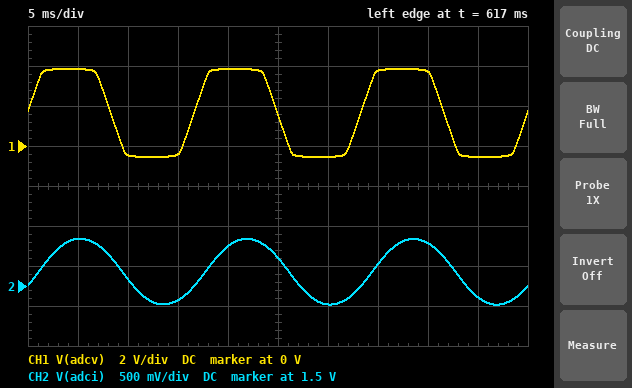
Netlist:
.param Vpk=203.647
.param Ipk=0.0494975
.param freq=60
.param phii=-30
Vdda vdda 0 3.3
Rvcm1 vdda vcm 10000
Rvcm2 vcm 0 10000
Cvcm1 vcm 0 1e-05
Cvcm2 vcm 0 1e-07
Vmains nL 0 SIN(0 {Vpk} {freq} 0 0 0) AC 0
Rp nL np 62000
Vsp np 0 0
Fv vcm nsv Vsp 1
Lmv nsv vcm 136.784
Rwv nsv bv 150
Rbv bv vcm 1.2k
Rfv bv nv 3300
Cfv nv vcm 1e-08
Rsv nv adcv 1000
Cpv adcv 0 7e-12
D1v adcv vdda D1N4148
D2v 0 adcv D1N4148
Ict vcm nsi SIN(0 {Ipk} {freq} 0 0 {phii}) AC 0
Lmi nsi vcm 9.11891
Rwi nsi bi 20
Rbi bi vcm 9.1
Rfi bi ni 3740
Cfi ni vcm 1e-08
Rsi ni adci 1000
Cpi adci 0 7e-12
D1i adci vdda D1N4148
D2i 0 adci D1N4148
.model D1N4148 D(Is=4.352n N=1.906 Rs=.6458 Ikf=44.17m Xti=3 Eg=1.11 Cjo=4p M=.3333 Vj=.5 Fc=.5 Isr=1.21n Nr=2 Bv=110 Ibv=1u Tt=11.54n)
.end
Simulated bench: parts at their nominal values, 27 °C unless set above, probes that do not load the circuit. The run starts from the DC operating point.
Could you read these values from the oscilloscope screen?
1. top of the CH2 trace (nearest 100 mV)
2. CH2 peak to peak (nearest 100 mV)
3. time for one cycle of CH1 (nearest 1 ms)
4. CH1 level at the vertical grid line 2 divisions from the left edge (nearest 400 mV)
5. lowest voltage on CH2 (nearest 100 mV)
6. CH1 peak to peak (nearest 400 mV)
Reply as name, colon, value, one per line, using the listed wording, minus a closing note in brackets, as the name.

top of the CH2 trace: 2.1 V
CH2 peak to peak: 800 mV
time for one cycle of CH1: 17 ms
CH1 level at the vertical grid line 2 divisions from the left edge: -400 mV
lowest voltage on CH2: 1.3 V
CH1 peak to peak: 4.4 V
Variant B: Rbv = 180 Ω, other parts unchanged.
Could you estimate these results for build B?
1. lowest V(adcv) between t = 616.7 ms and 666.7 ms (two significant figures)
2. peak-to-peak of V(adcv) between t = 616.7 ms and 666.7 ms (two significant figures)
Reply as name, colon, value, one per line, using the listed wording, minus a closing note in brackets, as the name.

lowest V(adcv) between t = 616.7 ms and 666.7 ms: 1.1 V
peak-to-peak of V(adcv) between t = 616.7 ms and 666.7 ms: 1.2 V
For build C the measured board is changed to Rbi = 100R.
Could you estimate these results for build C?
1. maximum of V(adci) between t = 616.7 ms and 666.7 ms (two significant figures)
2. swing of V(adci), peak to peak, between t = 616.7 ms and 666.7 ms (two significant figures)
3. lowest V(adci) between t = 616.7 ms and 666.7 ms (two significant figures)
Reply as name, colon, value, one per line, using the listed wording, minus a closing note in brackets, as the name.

maximum of V(adci) between t = 616.7 ms and 666.7 ms: 3.9 V
swing of V(adci), peak to peak, between t = 616.7 ms and 666.7 ms: 4.5 V
lowest V(adci) between t = 616.7 ms and 666.7 ms: -580 mV
